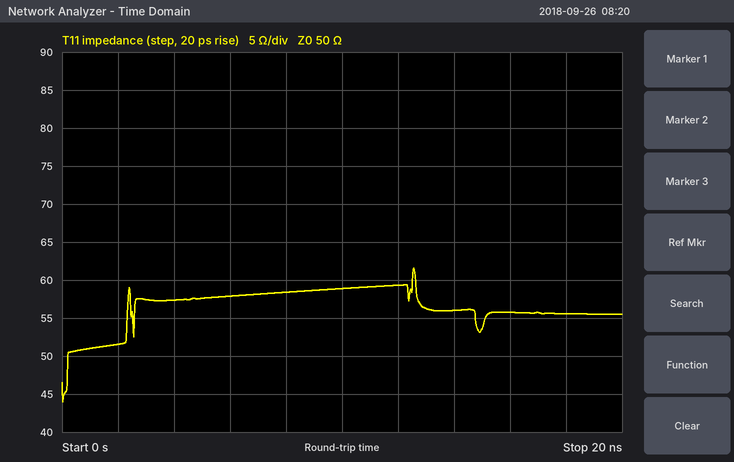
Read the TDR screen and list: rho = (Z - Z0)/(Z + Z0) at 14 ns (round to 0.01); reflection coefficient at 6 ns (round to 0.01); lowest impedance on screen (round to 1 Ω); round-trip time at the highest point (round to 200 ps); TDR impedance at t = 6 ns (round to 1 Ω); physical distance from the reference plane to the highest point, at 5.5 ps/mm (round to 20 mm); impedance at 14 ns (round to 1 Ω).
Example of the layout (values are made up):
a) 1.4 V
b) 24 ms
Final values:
a) +0.06
b) +0.07
c) 44 Ω
d) 12.6 ns
e) 58 Ω
f) 1.14 m
g) 56 Ω
